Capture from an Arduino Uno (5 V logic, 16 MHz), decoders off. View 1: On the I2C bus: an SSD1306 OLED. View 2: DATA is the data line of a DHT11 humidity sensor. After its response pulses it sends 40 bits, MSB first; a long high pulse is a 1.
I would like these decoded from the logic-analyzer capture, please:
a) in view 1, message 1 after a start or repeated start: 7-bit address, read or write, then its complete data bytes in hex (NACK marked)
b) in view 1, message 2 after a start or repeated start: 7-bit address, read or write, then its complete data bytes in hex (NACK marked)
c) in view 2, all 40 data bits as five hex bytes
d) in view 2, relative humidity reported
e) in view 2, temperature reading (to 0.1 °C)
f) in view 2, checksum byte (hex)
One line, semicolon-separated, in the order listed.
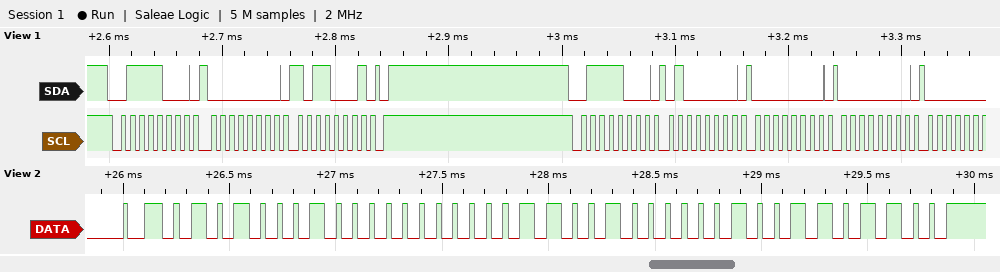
0x3C write: 00 B1; 0x3C write: 40 00 00; 51 00 19 02 6C; 81 %; 25.2 °C; 0x6C
